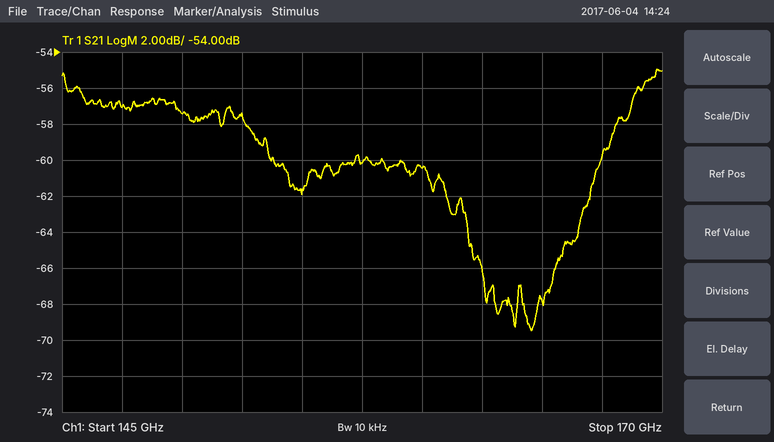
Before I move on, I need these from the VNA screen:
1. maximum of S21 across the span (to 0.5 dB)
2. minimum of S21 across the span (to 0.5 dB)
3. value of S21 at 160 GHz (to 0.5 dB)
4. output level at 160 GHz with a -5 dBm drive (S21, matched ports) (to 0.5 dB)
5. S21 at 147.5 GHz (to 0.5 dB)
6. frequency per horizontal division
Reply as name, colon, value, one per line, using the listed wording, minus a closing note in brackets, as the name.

maximum of S21 across the span: -55.0 dB
minimum of S21 across the span: -69.5 dB
value of S21 at 160 GHz: -60.5 dB
output level at 160 GHz with a -5 dBm drive (S21, matched ports): -65.5 dBm
S21 at 147.5 GHz: -57.0 dB
frequency per horizontal division: 2.5 GHz
